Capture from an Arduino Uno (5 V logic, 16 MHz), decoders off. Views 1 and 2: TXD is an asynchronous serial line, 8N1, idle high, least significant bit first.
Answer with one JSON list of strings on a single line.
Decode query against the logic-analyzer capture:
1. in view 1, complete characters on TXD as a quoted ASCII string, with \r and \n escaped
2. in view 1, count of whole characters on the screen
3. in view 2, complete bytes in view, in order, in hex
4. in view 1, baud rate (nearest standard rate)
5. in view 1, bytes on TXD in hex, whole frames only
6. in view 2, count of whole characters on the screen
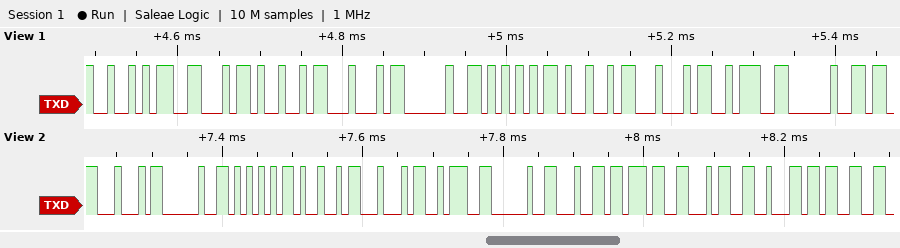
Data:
["\"RFID UID: \"", "10", "44 20 55 49 44 3A 20 64 37 34 62 33", "115200 baud", "52 46 49 44 20 55 49 44 3A 20", "12"]
